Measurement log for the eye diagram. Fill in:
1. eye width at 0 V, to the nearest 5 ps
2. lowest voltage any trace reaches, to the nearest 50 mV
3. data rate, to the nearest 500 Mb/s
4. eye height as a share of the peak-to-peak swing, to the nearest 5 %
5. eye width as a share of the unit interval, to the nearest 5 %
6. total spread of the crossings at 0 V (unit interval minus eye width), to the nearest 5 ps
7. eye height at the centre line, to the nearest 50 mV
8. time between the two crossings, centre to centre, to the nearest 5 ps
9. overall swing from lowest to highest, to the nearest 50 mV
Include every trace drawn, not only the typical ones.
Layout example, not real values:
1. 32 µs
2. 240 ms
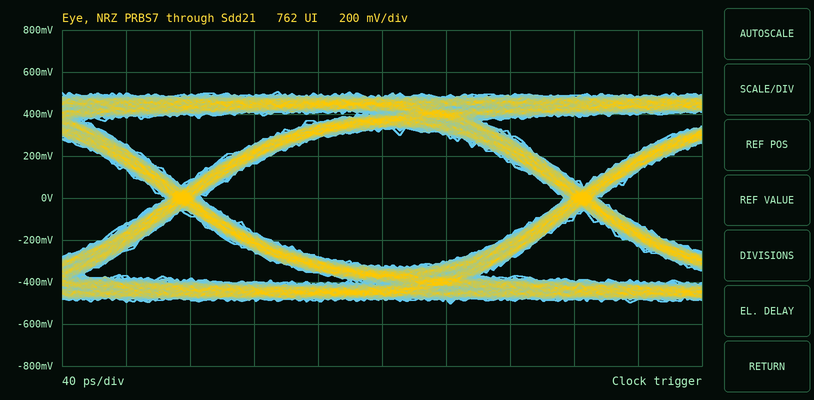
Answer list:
1. 225 ps
2. -500 mV
3. 4.0 Gb/s
4. 65 %
5. 90 %
6. 25 ps
7. 650 mV
8. 250 ps
9. 1.00 V
